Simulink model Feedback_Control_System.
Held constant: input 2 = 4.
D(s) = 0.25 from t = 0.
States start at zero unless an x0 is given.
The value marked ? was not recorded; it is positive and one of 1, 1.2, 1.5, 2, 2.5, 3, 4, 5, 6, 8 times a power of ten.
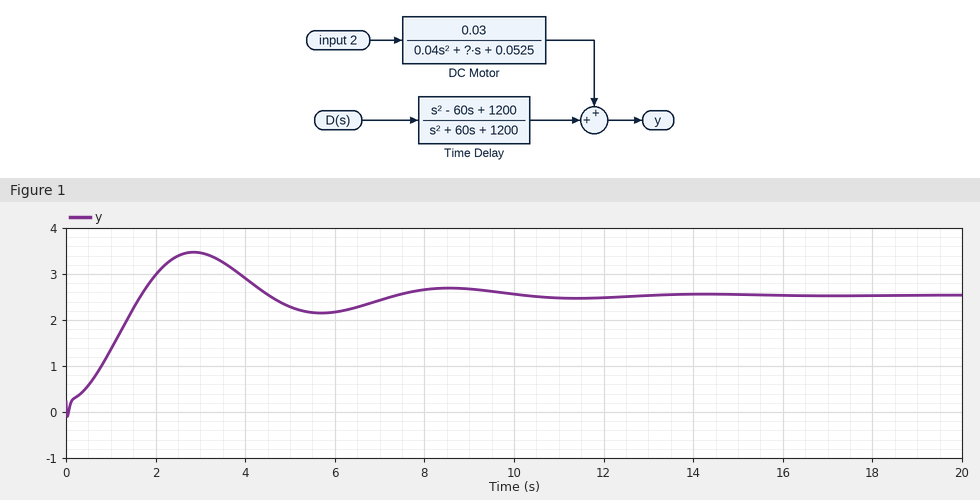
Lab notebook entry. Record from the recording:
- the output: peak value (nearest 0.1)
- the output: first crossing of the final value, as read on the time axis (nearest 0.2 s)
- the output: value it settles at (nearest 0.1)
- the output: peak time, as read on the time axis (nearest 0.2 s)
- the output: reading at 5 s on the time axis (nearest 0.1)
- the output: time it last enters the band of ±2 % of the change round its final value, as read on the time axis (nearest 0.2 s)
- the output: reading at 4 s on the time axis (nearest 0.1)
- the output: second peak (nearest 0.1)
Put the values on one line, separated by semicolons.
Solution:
3.5; 1.6 s; 2.5; 2.8 s; 2.3; 12.2 s; 2.9; 2.7
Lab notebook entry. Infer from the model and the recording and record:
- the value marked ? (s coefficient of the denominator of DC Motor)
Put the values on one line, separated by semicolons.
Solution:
0.025
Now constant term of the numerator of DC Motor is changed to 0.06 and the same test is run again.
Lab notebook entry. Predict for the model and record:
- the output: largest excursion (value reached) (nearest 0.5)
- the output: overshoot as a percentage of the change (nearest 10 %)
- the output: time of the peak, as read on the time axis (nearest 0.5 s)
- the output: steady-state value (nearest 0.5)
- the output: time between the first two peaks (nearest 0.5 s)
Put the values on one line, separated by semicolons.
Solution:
6.5; 40 %; 3.0 s; 5.0; 5.5 s
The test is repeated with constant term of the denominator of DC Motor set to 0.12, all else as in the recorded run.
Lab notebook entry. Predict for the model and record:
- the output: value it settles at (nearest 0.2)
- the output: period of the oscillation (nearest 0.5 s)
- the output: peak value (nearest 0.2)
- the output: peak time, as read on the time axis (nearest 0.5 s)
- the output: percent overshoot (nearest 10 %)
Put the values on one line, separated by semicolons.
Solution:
1.2; 3.5 s; 1.8; 2.0 s; 60 %
